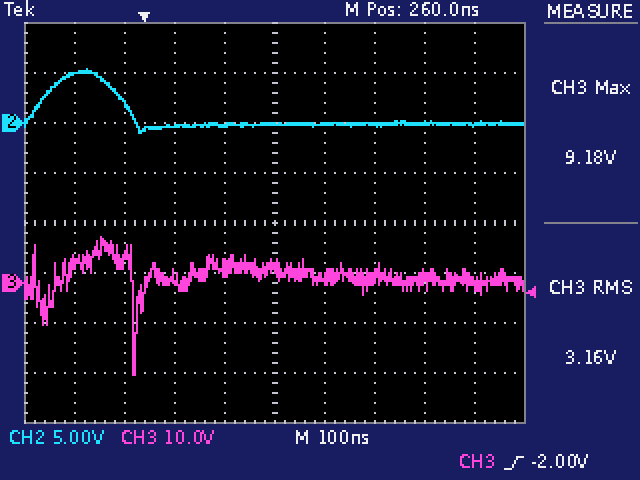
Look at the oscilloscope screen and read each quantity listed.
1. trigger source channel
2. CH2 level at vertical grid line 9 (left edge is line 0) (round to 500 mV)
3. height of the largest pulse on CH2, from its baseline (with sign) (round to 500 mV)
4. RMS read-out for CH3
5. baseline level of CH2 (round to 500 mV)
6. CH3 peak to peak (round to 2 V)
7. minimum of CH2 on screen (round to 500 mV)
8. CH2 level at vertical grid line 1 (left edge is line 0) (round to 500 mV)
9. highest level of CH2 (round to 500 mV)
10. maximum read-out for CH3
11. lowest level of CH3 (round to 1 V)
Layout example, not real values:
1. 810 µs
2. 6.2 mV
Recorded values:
1. CH3
2. 0.0 V
3. +5.5 V
4. 3.16 V
5. 0.0 V
6. 28 V
7. -1.0 V
8. 5.0 V
9. 5.5 V
10. 9.18 V
11. -18 V
